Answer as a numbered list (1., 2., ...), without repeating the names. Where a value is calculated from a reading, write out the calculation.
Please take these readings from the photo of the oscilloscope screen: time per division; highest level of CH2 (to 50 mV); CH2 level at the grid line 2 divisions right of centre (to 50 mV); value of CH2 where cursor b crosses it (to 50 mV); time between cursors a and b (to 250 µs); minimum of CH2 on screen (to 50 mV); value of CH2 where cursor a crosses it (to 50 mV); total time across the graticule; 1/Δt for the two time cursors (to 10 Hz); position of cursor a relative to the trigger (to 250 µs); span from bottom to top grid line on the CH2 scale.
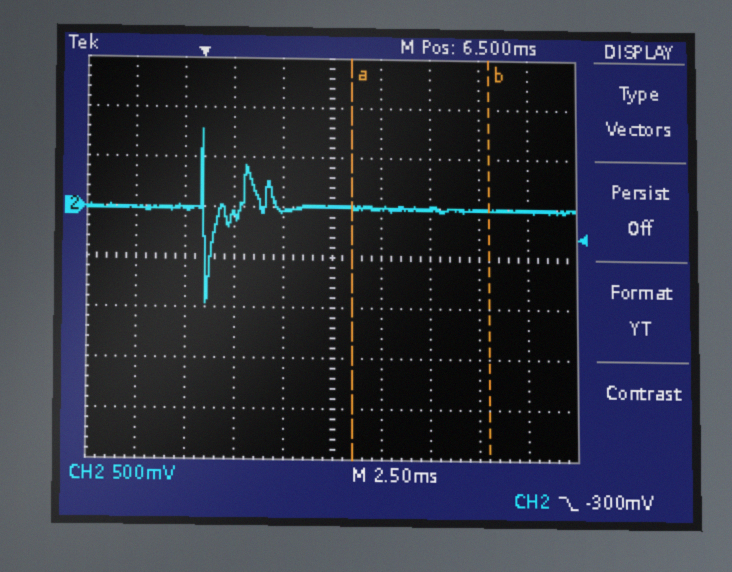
1. 2.5 ms
2. 800 mV
3. 0 mV
4. 0 mV
5. 7.00 ms
6. -950 mV
7. 0 mV
8. 25 ms
9. 1 / 7.00 ms ≈ 140 Hz
10. +7.50 ms
11. 4 V
